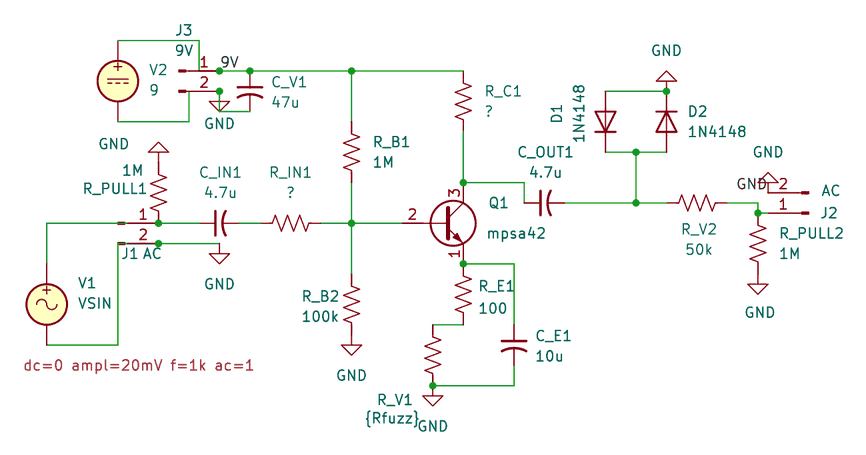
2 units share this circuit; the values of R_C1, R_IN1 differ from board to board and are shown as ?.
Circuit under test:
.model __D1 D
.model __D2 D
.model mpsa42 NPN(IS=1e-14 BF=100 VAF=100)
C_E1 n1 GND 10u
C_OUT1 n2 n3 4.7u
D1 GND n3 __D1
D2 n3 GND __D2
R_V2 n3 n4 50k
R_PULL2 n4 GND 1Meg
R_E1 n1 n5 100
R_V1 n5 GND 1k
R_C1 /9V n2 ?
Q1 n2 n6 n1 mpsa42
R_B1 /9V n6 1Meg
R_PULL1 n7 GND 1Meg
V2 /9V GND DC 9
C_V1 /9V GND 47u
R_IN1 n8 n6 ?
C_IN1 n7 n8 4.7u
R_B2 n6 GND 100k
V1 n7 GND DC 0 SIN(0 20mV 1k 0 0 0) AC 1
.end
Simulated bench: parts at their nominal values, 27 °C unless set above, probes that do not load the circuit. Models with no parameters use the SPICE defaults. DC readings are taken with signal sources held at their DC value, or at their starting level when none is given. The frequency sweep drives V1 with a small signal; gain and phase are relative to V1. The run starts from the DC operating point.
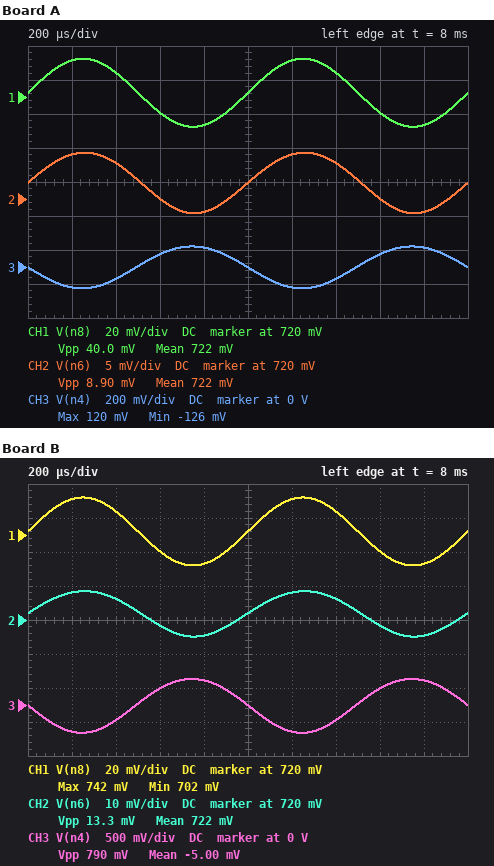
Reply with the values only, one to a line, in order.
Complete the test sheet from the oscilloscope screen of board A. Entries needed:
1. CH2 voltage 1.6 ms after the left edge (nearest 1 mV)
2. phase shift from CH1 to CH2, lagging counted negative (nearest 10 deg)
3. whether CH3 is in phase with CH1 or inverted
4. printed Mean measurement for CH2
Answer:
720 mV
0 deg
inverted
722 mV
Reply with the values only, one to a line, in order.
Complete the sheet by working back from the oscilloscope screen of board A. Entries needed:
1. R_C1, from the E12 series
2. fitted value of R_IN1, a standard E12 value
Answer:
6.8 kΩ
68 kΩ
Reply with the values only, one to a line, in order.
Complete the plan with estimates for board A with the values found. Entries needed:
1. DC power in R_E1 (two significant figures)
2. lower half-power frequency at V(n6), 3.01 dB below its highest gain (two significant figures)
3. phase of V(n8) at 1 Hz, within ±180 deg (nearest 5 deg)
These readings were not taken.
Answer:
1.3 µW
270 mHz
15 deg
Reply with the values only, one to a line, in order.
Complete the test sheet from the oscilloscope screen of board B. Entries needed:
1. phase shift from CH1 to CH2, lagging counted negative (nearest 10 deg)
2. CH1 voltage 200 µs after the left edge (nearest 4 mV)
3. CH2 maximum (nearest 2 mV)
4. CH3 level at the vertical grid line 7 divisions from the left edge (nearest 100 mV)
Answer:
0 deg
740 mV
728 mV
-200 mV
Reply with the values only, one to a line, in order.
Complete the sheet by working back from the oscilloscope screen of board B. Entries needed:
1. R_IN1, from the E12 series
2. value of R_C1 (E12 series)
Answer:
39 kΩ
15 kΩ
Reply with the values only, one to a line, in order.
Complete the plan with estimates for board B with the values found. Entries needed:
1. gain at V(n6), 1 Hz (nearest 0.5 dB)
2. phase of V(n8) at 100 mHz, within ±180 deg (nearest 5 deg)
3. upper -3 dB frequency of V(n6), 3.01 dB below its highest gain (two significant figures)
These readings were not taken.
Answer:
-5.0 dB
75 deg
81 Hz
